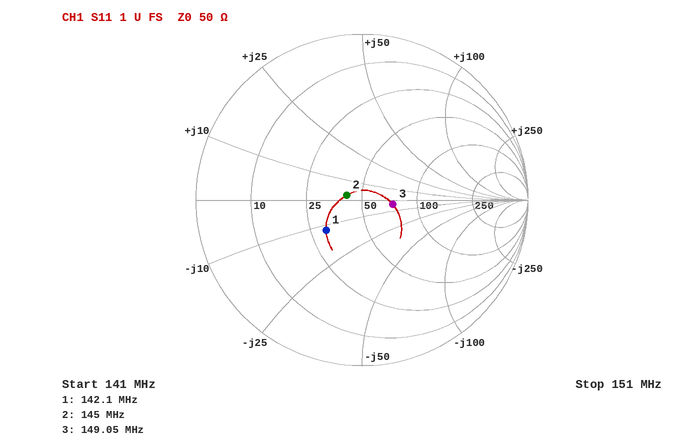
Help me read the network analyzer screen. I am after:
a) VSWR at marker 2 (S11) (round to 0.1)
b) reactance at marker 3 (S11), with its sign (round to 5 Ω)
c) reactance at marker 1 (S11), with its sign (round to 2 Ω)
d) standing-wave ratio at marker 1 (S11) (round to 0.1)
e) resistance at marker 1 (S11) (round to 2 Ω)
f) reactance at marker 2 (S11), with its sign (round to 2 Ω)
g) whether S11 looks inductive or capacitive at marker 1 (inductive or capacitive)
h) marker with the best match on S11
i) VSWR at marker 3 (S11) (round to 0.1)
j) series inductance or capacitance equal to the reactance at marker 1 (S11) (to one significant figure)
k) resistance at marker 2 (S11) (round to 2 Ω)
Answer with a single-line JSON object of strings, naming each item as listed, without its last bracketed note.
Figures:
{"VSWR at marker 2 (S11)": "1.2", "reactance at marker 3 (S11), with its sign": "-5 Ω", "reactance at marker 1 (S11), with its sign": "-12 Ω", "standing-wave ratio at marker 1 (S11)": "1.8", "resistance at marker 1 (S11)": "30 Ω", "reactance at marker 2 (S11), with its sign": "+2 Ω", "whether S11 looks inductive or capacitive at marker 1": "capacitive", "marker with the best match on S11": "marker 2", "VSWR at marker 3 (S11)": "1.5", "series inductance or capacitance equal to the reactance at marker 1 (S11)": "90 pF", "resistance at marker 2 (S11)": "42 Ω"}
